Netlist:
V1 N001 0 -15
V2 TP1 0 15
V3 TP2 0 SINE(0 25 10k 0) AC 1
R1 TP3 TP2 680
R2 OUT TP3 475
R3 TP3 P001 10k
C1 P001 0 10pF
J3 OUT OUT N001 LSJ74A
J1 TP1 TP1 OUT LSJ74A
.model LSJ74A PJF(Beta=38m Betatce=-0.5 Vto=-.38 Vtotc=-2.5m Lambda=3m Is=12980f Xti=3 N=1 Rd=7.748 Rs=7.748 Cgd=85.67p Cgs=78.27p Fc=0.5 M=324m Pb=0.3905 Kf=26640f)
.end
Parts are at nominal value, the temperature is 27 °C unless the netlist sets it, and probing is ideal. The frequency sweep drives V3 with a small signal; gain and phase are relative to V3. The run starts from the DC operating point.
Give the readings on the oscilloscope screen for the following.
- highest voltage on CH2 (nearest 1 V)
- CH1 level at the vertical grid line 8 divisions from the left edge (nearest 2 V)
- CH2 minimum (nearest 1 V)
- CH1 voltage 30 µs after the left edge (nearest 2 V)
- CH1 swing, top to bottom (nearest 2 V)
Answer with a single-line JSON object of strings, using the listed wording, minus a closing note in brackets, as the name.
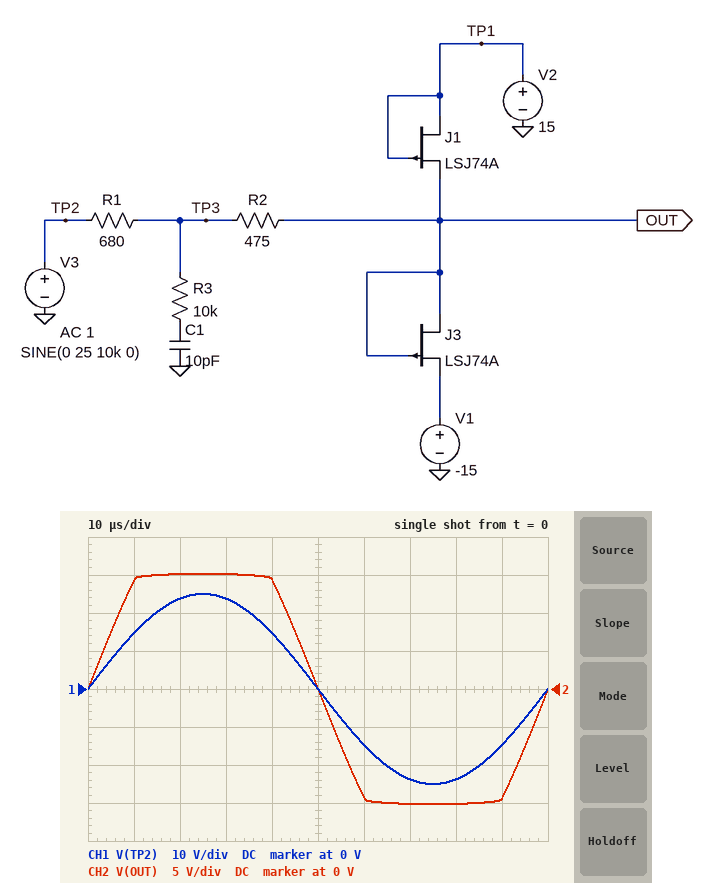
{"highest voltage on CH2": "15 V", "CH1 level at the vertical grid line 8 divisions from the left edge": "-24 V", "CH2 minimum": "-15 V", "CH1 voltage 30 µs after the left edge": "24 V", "CH1 swing, top to bottom": "50 V"}
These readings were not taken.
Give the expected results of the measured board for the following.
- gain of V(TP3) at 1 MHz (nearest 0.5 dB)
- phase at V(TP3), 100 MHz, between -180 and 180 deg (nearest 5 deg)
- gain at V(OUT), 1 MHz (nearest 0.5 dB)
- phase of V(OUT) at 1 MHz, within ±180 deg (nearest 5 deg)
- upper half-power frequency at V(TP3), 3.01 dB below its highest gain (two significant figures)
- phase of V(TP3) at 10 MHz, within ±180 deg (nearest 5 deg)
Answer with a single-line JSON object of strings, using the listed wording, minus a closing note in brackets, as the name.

{"gain of V(TP3) at 1 MHz": "-0.5 dB", "phase at V(TP3), 100 MHz, between -180 and 180 deg": "-5 deg", "gain at V(OUT), 1 MHz": "-0.5 dB", "phase of V(OUT) at 1 MHz, within ±180 deg": "-10 deg", "upper half-power frequency at V(TP3), 3.01 dB below its highest gain": "6.2 MHz", "phase of V(TP3) at 10 MHz, within ±180 deg": "-25 deg"}
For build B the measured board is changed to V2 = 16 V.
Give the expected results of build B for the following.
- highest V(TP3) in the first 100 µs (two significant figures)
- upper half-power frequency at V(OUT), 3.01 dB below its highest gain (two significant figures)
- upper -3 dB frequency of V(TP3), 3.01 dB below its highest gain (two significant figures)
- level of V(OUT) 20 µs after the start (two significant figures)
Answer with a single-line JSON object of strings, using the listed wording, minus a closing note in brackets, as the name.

{"highest V(TP3) in the first 100 µs": "20 V", "upper half-power frequency at V(OUT), 3.01 dB below its highest gain": "5.2 MHz", "upper -3 dB frequency of V(TP3), 3.01 dB below its highest gain": "6.3 MHz", "level of V(OUT) 20 µs after the start": "16 V"}
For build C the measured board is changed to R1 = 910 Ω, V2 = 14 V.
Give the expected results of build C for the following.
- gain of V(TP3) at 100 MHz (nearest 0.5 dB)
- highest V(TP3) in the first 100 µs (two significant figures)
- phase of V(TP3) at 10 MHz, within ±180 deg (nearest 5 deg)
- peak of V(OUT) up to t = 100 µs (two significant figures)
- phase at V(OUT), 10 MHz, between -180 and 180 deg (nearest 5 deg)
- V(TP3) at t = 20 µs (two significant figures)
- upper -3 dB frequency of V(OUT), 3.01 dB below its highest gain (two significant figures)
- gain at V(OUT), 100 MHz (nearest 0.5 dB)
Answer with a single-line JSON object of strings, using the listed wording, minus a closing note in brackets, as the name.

{"gain of V(TP3) at 100 MHz": "-9.5 dB", "highest V(TP3) in the first 100 µs": "18 V", "phase of V(TP3) at 10 MHz, within ±180 deg": "-25 deg", "peak of V(OUT) up to t = 100 µs": "14 V", "phase at V(OUT), 10 MHz, between -180 and 180 deg": "-65 deg", "V(TP3) at t = 20 µs": "17 V", "upper -3 dB frequency of V(OUT), 3.01 dB below its highest gain": "4.1 MHz", "gain at V(OUT), 100 MHz": "-27.0 dB"}
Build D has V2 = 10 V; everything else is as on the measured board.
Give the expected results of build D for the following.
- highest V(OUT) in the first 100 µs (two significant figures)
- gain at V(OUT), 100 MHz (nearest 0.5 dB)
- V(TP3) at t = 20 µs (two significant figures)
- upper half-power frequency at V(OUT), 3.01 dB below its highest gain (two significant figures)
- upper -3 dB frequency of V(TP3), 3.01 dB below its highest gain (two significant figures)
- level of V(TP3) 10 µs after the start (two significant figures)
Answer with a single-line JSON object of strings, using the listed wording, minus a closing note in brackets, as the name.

{"highest V(OUT) in the first 100 µs": "10 V", "gain at V(OUT), 100 MHz": "-26.5 dB", "V(TP3) at t = 20 µs": "16 V", "upper half-power frequency at V(OUT), 3.01 dB below its highest gain": "4.6 MHz", "upper -3 dB frequency of V(TP3), 3.01 dB below its highest gain": "5.6 MHz", "level of V(TP3) 10 µs after the start": "12 V"}
